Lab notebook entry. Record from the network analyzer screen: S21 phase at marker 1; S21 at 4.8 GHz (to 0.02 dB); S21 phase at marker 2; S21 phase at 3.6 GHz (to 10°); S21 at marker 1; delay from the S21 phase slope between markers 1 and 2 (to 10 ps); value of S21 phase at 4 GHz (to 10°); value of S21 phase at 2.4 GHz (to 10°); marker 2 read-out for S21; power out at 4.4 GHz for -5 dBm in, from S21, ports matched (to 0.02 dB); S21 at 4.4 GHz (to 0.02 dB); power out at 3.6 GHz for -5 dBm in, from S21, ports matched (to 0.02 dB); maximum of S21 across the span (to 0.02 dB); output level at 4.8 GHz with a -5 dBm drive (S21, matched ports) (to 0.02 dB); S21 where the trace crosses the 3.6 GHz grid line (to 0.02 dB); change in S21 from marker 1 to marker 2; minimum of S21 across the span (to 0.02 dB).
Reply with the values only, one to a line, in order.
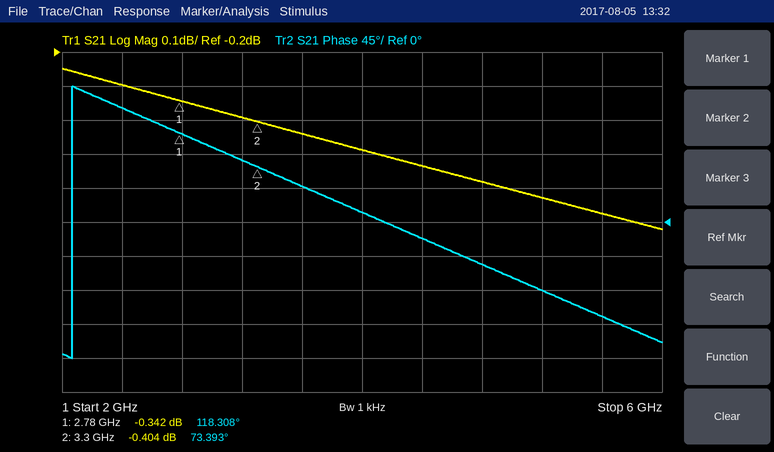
118.308°
-0.58 dB
73.393°
50°
-0.342 dB
240 ps
10°
150°
-0.404 dB
-5.54 dBm
-0.54 dB
-5.44 dBm
-0.24 dB
-5.58 dBm
-0.44 dB
-0.062 dB
-0.72 dB
